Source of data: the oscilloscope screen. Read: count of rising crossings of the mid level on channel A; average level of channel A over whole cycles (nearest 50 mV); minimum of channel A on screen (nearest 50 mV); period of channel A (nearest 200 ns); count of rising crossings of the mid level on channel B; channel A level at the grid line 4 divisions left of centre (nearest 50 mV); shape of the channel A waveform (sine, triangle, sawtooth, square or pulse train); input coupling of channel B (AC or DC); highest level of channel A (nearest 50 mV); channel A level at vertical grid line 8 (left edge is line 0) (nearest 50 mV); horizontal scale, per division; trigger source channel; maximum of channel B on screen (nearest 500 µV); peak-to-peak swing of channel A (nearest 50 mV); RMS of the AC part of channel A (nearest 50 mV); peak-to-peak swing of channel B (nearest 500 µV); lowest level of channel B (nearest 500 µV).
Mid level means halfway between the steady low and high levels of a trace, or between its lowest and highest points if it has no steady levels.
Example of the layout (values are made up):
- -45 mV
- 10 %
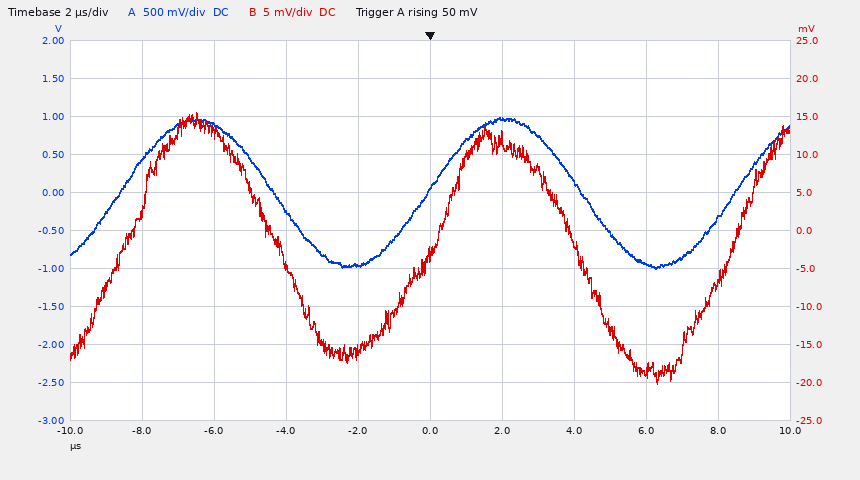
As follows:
- 3
- 0 mV
- -1.00 V
- 8.6 µs
- 3
- 450 mV
- sine
- DC
- 1.00 V
- -950 mV
- 2 µs
- channel A
- 15.5 mV
- 2.00 V
- 700 mV
- 35.5 mV
- -20.0 mV
